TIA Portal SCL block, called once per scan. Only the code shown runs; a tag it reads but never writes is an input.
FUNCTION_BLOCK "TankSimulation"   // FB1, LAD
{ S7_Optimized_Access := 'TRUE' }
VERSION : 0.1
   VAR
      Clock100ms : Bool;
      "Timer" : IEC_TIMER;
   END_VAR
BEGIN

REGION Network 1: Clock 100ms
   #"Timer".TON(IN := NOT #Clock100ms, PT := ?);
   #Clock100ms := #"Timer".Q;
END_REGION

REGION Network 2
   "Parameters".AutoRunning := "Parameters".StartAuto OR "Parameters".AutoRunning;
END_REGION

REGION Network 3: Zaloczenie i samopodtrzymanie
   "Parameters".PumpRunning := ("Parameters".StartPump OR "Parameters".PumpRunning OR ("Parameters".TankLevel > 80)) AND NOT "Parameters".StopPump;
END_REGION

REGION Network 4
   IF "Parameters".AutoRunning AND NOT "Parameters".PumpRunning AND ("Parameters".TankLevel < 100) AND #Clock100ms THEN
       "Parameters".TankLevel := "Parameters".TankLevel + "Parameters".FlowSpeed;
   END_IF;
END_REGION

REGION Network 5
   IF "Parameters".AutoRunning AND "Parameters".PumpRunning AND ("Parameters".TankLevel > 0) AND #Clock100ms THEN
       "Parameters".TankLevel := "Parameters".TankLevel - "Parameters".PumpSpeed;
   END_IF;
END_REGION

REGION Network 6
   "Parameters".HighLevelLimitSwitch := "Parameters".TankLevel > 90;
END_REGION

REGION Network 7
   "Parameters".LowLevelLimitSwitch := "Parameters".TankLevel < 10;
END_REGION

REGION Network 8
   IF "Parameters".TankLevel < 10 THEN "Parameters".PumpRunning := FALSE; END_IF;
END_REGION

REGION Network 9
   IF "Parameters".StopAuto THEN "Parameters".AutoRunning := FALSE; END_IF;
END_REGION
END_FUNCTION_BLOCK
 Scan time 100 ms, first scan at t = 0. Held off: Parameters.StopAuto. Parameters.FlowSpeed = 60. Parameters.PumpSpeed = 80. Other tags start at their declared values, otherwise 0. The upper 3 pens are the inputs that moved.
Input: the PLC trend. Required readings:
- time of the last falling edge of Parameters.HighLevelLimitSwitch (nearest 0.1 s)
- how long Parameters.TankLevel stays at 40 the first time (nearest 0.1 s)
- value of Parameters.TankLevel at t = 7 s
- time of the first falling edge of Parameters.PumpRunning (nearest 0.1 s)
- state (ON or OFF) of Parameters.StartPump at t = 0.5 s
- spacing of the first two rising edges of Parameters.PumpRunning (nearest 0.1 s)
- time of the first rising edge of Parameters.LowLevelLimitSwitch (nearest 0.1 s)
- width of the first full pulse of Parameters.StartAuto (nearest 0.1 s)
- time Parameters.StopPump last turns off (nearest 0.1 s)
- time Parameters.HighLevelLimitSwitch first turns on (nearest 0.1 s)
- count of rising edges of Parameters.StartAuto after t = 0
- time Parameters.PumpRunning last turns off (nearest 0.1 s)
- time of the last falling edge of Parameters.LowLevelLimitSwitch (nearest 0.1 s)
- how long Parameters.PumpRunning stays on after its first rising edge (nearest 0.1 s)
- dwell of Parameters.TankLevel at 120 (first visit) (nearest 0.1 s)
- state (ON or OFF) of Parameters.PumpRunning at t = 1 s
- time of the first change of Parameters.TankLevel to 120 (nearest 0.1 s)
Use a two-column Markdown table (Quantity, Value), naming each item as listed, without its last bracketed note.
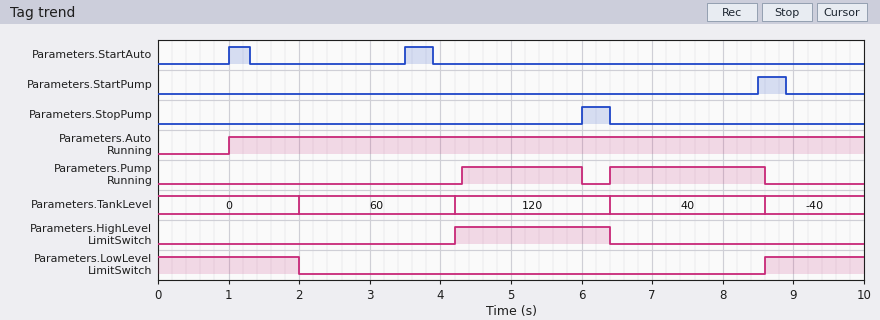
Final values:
| Quantity | Value |
|---|---|
| time of the last falling edge of Parameters.HighLevelLimitSwitch | 6.4 s |
| how long Parameters.TankLevel stays at 40 the first time | 2.2 s |
| value of Parameters.TankLevel at t = 7 s | 40 |
| time of the first falling edge of Parameters.PumpRunning | 6.0 s |
| state (ON or OFF) of Parameters.StartPump at t = 0.5 s | OFF |
| spacing of the first two rising edges of Parameters.PumpRunning | 2.1 s |
| time of the first rising edge of Parameters.LowLevelLimitSwitch | 8.6 s |
| width of the first full pulse of Parameters.StartAuto | 0.3 s |
| time Parameters.StopPump last turns off | 6.4 s |
| time Parameters.HighLevelLimitSwitch first turns on | 4.2 s |
| count of rising edges of Parameters.StartAuto after t = 0 | 2 |
| time Parameters.PumpRunning last turns off | 8.6 s |
| time of the last falling edge of Parameters.LowLevelLimitSwitch | 2.0 s |
| how long Parameters.PumpRunning stays on after its first rising edge | 1.7 s |
| dwell of Parameters.TankLevel at 120 (first visit) | 2.2 s |
| state (ON or OFF) of Parameters.PumpRunning at t = 1 s | OFF |
| time of the first change of Parameters.TankLevel to 120 | 4.2 s |
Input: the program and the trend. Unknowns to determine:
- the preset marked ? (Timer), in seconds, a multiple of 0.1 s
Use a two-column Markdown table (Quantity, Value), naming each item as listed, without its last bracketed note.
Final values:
| Quantity | Value |
|---|---|
| the preset marked ? (Timer), in seconds, a multiple of 0.1 s | 2.0 s |
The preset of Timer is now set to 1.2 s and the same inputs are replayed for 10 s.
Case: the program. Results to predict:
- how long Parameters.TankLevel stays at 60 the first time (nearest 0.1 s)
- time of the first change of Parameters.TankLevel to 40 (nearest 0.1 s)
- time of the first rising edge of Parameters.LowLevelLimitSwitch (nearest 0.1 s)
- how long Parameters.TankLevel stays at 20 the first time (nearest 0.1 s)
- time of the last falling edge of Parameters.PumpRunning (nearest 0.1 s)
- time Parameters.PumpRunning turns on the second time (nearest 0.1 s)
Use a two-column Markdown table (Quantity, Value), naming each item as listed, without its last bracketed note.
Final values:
| Quantity | Value |
|---|---|
| how long Parameters.TankLevel stays at 60 the first time | 1.4 s |
| time of the first change of Parameters.TankLevel to 40 | 4.0 s |
| time of the first rising edge of Parameters.LowLevelLimitSwitch | 5.4 s |
| how long Parameters.TankLevel stays at 20 the first time | 1.4 s |
| time of the last falling edge of Parameters.PumpRunning | 9.6 s |
| time Parameters.PumpRunning turns on the second time | 8.5 s |
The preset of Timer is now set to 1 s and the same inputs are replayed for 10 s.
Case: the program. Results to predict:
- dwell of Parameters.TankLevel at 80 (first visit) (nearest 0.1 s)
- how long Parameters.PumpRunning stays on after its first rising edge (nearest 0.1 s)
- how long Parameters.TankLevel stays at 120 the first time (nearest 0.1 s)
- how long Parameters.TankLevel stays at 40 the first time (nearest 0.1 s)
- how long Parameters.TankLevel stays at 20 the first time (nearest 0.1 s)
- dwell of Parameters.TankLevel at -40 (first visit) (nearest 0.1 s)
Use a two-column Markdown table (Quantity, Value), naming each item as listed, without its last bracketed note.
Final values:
| Quantity | Value |
|---|---|
| dwell of Parameters.TankLevel at 80 (first visit) | 1.2 s |
| how long Parameters.PumpRunning stays on after its first rising edge | 2.3 s |
| how long Parameters.TankLevel stays at 120 the first time | 1.2 s |
| how long Parameters.TankLevel stays at 40 the first time | 1.2 s |
| how long Parameters.TankLevel stays at 20 the first time | 1.2 s |
| dwell of Parameters.TankLevel at -40 (first visit) | 1.2 s |
